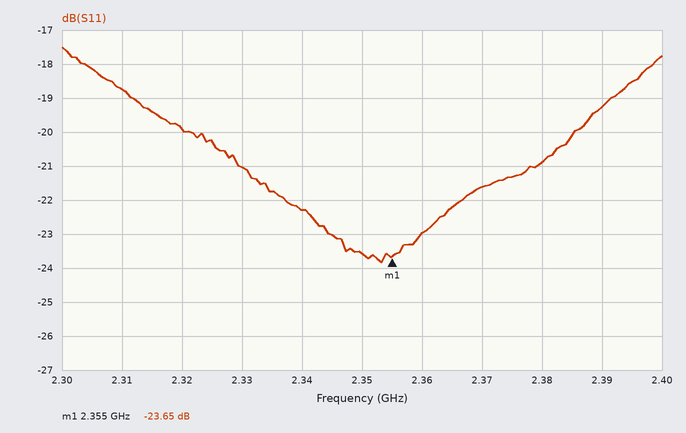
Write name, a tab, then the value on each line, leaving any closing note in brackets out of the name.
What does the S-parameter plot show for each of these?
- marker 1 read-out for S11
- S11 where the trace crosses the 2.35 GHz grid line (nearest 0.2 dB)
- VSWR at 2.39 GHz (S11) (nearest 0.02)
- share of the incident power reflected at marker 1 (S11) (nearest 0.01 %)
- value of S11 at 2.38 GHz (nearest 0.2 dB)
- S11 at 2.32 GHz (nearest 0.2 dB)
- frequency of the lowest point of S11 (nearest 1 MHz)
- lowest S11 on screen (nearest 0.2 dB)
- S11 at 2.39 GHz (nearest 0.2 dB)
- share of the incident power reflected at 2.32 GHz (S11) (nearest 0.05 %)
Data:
marker 1 read-out for S11	-23.65 dB
S11 where the trace crosses the 2.35 GHz grid line	-23.6 dB
VSWR at 2.39 GHz (S11)	1.24
share of the incident power reflected at marker 1 (S11)	0.43 %
value of S11 at 2.38 GHz	-20.8 dB
S11 at 2.32 GHz	-20.0 dB
frequency of the lowest point of S11	2.353 GHz
lowest S11 on screen	-23.8 dB
S11 at 2.39 GHz	-19.2 dB
share of the incident power reflected at 2.32 GHz (S11)	1.00 %
